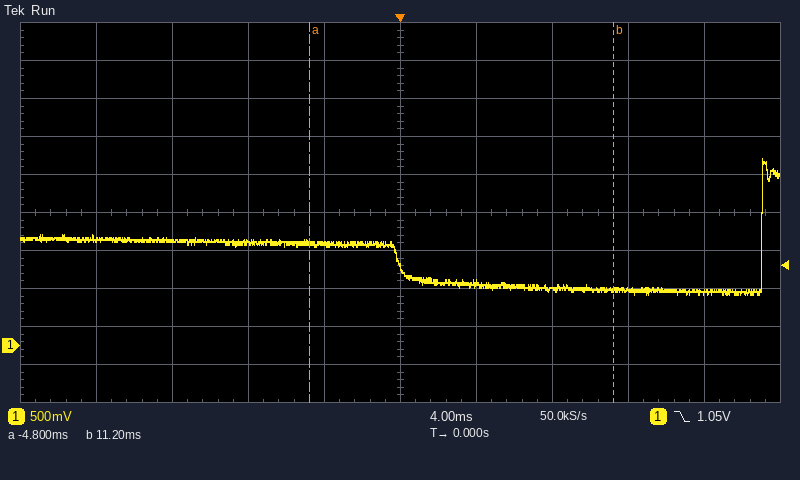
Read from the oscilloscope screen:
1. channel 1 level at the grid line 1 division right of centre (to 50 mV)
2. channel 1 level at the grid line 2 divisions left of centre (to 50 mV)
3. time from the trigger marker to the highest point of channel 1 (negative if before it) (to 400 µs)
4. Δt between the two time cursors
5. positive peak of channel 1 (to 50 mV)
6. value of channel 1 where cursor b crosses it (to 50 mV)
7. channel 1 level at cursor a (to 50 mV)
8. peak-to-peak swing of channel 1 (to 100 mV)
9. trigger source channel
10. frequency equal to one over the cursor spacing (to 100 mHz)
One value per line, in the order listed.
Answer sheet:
800 mV
1.35 V
+19.2 ms
16.0 ms
2.45 V
750 mV
1.35 V
1.80 V
channel 1
62.5 Hz
